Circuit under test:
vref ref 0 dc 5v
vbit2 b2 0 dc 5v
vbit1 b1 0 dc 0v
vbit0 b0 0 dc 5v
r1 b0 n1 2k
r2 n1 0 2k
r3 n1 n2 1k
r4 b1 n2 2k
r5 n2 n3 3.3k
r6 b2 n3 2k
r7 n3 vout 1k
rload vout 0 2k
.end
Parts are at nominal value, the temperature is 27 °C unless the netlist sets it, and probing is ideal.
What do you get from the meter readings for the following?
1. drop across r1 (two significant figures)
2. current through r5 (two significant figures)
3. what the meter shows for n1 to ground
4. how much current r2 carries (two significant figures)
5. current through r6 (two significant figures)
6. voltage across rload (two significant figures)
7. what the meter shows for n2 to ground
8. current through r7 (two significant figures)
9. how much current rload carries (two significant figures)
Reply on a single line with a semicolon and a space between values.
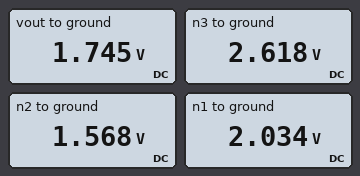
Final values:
3.0 V; 320 µA; 2.034 V; 1.0 mA; 1.2 mA; 1.7 V; 1.568 V; 870 µA; 870 µA
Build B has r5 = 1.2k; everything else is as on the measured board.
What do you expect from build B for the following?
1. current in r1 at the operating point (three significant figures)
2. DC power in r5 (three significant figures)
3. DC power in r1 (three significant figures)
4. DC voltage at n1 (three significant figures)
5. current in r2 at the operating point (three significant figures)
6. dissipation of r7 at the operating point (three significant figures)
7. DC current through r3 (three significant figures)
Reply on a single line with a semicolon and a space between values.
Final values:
1.43 mA; 318 µW; 4.11 mW; 2.13 V; 1.07 mA; 631 µW; 368 µA
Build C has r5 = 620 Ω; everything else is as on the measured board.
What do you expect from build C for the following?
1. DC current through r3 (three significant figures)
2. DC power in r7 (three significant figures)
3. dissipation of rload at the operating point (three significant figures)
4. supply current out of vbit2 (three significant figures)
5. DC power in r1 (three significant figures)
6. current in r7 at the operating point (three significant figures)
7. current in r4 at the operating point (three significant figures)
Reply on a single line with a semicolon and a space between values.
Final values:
315 µA; 565 µW; 1.13 mW; 1.37 mA; 3.96 mW; 752 µA; 935 µA
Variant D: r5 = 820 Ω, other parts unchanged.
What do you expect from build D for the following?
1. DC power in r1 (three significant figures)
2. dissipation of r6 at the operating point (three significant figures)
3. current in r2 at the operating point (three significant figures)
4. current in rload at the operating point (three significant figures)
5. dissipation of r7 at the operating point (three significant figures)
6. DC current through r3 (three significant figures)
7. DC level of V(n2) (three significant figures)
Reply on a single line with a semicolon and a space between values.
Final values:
4.02 mW; 3.63 mW; 1.08 mA; 768 µA; 590 µW; 335 µA; 1.83 V
